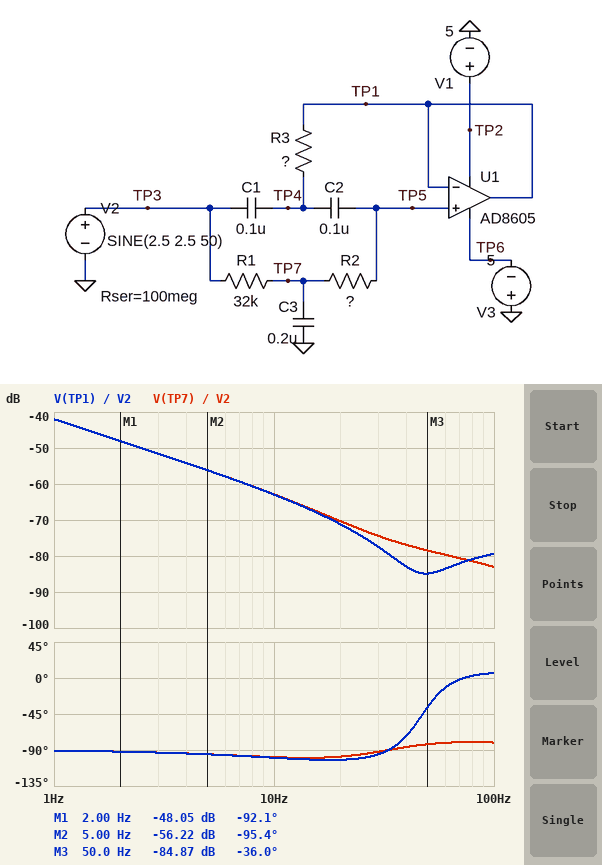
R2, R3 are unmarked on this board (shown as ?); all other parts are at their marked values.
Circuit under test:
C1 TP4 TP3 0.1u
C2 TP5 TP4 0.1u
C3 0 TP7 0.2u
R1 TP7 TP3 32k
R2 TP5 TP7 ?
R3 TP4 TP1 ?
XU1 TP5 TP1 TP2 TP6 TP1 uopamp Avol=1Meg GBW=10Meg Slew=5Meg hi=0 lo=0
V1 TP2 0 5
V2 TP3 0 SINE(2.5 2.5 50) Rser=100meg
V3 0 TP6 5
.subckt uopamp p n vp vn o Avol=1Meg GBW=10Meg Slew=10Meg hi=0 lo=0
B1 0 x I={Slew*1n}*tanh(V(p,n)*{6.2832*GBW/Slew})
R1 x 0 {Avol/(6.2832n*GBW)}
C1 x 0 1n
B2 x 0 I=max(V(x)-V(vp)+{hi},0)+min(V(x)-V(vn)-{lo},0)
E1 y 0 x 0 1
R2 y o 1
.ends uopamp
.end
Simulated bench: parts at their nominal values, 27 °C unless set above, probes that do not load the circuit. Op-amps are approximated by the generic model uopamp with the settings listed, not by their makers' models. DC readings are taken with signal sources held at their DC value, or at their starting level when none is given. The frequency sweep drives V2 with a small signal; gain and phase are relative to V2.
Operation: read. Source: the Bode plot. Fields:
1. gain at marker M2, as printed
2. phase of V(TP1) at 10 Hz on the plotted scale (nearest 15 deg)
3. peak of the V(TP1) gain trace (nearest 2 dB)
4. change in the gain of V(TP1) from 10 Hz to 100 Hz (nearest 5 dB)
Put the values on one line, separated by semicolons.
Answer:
-56.22 dB; -105 deg; -42 dB; -15 dB
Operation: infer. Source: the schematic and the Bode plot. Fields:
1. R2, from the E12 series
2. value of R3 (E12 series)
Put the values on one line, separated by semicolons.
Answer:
27 kΩ; 39 kΩ
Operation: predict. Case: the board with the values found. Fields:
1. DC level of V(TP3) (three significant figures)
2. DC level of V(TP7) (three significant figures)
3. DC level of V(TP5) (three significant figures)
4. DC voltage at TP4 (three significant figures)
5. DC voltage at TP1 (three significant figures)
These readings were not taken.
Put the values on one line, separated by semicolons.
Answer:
2.50 V; 2.50 V; 2.50 V; 2.50 V; 2.50 V
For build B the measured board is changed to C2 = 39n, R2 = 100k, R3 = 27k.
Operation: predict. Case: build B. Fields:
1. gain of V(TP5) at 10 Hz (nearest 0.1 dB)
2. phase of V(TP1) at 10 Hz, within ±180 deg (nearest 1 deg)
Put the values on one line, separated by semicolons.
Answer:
-62.6 dB; -102 deg
